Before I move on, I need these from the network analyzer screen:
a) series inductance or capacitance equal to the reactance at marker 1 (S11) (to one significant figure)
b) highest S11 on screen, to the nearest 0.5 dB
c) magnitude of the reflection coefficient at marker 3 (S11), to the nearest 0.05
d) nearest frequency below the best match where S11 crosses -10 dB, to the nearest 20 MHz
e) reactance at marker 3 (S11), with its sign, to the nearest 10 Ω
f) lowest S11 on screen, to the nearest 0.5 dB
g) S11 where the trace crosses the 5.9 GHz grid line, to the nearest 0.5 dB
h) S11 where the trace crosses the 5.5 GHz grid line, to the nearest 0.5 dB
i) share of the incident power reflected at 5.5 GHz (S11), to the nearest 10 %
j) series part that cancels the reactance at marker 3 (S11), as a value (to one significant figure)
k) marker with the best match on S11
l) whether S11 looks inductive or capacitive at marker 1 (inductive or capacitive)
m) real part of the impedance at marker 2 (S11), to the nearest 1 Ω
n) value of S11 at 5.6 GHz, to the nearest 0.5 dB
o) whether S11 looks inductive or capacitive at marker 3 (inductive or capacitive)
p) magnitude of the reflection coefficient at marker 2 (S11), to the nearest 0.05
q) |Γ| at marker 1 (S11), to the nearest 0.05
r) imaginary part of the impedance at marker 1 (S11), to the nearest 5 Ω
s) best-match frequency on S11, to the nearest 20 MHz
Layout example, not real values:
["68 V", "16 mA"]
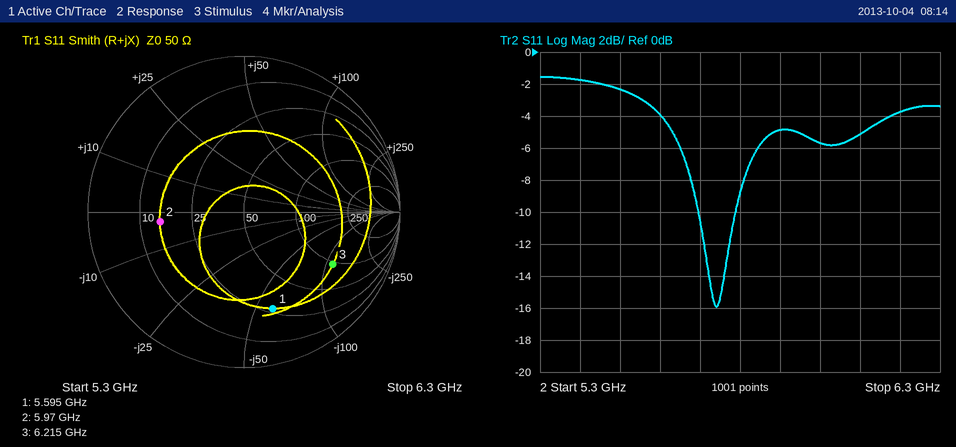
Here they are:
["500 fF", "-1.5 dB", "0.65", "5.70 GHz", "-110 Ω", "-16.0 dB", "-5.0 dB", "-2.5 dB", "60 %", "3 nH", "marker 2", "capacitive", "15 Ω", "-4.0 dB", "capacitive", "0.55", "0.65", "-60 Ω", "5.74 GHz"]
